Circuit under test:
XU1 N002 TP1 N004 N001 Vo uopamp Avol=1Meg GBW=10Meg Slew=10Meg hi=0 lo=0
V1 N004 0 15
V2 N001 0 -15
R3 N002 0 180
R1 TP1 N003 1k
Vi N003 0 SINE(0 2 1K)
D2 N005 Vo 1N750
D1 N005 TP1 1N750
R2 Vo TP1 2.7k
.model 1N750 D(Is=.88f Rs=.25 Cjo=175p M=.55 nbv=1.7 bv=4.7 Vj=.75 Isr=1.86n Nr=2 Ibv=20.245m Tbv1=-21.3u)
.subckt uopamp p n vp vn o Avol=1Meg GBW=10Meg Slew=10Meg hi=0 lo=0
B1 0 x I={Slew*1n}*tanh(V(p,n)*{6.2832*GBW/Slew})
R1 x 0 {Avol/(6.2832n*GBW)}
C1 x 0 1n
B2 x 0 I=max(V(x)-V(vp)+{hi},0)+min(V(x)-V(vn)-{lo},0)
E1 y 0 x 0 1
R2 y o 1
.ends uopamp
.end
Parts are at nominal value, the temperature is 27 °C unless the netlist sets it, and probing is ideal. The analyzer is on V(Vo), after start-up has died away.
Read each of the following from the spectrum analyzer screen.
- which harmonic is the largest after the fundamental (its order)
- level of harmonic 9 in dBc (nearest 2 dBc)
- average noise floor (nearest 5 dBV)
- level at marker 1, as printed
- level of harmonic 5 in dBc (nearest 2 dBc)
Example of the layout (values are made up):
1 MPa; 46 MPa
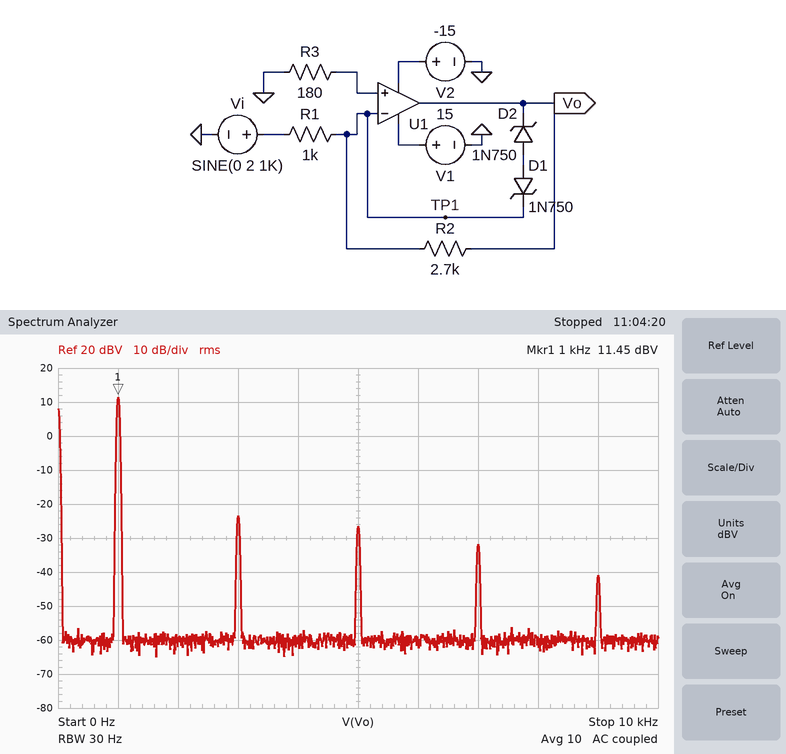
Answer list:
3; -52 dBc; -60 dBV; 11.45 dBV; -38 dBc
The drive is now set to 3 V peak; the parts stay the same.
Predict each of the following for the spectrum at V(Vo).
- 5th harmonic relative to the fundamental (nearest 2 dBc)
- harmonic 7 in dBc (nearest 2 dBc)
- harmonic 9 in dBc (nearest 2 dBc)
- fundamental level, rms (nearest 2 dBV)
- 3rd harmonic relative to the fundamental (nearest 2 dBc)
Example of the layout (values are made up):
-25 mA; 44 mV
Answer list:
-44 dBc; -32 dBc; -50 dBc; 12 dBV; -16 dBc
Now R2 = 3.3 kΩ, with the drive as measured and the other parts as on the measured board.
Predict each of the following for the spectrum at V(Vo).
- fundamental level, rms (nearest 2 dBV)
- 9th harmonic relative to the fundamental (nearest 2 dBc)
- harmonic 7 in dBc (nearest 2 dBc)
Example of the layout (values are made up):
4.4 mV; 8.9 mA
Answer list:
12 dBV; -42 dBc; -46 dBc
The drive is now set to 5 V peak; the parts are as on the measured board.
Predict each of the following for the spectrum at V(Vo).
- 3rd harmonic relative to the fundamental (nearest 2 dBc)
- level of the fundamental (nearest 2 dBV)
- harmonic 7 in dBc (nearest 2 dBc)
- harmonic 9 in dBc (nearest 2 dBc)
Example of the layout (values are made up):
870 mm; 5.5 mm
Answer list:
-12 dBc; 14 dBV; -34 dBc; -40 dBc
